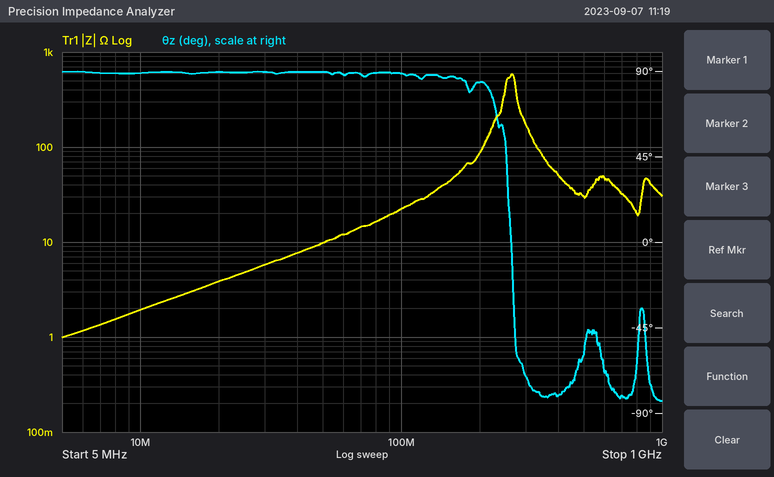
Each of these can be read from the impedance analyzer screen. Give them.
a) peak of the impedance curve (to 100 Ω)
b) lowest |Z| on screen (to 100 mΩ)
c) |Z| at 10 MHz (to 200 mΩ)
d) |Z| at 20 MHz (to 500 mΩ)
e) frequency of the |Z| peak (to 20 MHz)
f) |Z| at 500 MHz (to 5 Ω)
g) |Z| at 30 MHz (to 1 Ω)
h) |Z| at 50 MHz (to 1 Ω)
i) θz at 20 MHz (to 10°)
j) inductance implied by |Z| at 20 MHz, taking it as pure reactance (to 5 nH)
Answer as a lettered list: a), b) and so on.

a) 600 Ω
b) 1.0 Ω
c) 2.0 Ω
d) 4.0 Ω
e) 260 MHz
f) 30 Ω
g) 6 Ω
h) 10 Ω
i) 90°
j) 30 nH
